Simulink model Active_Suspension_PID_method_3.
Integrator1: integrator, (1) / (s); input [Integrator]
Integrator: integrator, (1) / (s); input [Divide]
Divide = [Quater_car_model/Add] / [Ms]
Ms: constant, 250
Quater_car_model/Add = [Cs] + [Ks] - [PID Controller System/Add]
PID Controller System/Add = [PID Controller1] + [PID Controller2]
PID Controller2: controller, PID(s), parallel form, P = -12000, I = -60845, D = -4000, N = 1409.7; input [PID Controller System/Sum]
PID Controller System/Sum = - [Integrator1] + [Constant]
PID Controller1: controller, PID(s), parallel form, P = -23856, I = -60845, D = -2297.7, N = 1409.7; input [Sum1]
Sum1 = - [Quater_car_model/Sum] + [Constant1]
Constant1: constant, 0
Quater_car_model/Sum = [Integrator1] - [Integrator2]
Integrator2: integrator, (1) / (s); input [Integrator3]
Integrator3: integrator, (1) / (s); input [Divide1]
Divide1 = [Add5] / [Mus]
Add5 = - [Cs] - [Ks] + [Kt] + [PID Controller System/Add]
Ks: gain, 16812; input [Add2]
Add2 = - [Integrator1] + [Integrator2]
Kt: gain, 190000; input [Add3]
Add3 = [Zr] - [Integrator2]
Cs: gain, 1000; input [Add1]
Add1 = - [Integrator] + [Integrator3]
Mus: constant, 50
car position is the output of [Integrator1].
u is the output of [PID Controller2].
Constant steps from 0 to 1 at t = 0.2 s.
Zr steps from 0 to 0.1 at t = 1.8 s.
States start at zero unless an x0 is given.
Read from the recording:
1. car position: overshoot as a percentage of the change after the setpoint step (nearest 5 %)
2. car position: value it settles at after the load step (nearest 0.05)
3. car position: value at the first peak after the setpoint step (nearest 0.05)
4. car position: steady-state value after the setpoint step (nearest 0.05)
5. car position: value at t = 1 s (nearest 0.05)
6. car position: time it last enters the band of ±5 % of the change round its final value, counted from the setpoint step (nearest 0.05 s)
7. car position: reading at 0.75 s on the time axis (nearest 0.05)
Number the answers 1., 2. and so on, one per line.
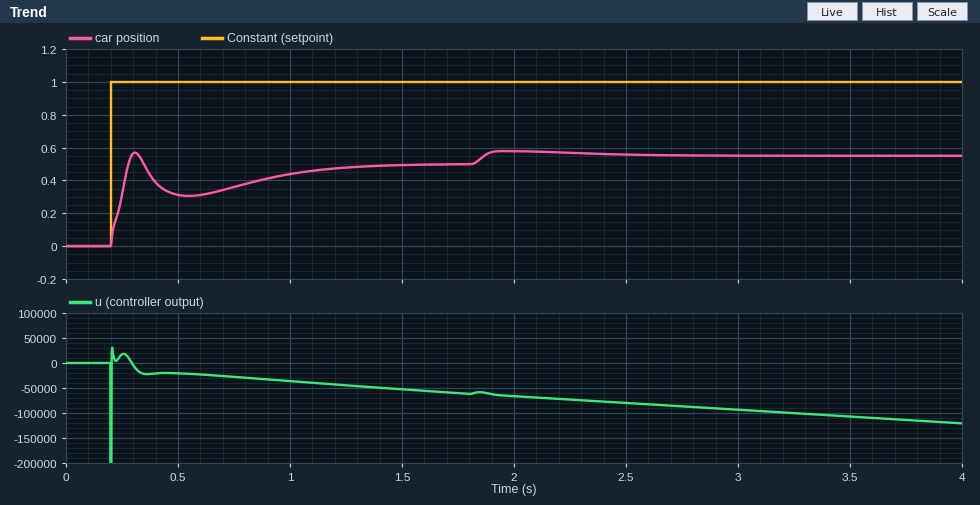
1. 15 %
2. 0.55
3. 0.55
4. 0.50
5. 0.45
6. 1.00 s
7. 0.35
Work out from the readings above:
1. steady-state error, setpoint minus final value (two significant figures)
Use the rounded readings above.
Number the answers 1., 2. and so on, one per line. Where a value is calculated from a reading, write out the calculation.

1. 1 - 0.5 = 0.50
